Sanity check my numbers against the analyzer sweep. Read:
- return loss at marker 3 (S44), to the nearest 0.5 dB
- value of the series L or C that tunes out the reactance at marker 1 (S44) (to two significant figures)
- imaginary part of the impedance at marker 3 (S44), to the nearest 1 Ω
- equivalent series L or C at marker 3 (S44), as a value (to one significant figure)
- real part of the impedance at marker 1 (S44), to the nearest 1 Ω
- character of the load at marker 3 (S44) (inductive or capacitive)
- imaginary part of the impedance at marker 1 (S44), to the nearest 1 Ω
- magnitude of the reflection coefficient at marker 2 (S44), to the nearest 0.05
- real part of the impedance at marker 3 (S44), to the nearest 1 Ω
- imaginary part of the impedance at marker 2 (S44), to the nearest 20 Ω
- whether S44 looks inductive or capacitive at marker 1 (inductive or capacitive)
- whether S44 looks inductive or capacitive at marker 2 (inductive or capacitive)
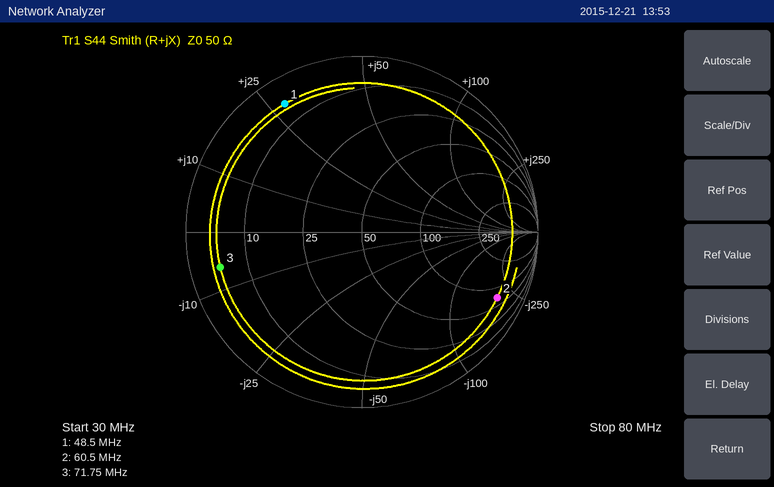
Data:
1.5 dB
120 pF
-6 Ω
400 pF
5 Ω
capacitive
+28 Ω
0.85
5 Ω
-200 Ω
inductive
capacitive
